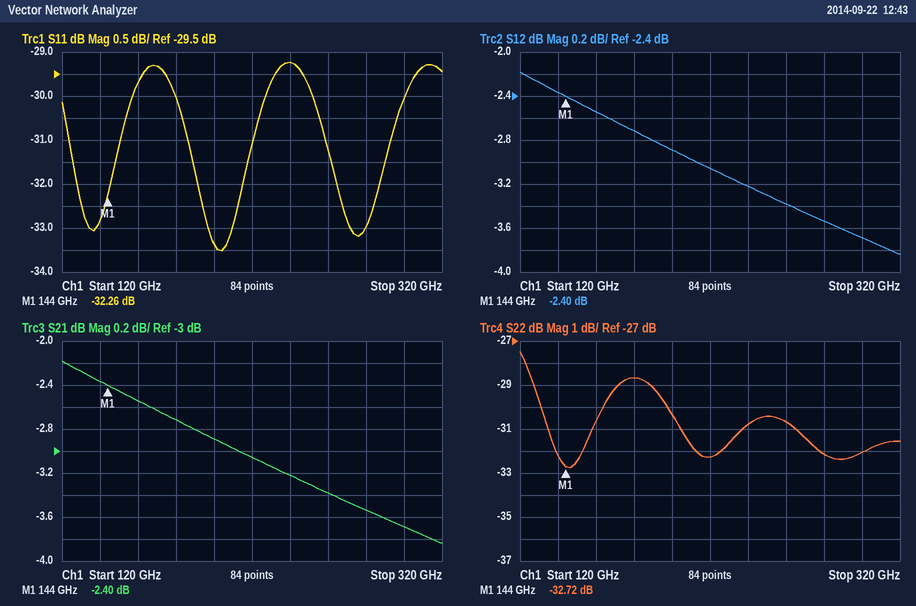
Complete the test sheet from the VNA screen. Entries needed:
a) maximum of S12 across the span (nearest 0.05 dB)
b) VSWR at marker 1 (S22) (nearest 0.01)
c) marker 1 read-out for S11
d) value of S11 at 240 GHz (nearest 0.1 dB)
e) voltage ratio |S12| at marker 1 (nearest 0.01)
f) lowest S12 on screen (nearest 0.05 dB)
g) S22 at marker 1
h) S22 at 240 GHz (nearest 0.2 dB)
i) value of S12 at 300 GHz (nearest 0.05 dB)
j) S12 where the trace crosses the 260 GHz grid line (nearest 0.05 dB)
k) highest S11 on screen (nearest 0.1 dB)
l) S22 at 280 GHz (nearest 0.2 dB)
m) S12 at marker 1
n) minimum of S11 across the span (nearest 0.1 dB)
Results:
-2.20 dB
1.05
-32.26 dB
-29.2 dB
0.76
-3.85 dB
-32.72 dB
-30.8 dB
-3.70 dB
-3.40 dB
-29.2 dB
-32.2 dB
-2.40 dB
-33.5 dB
